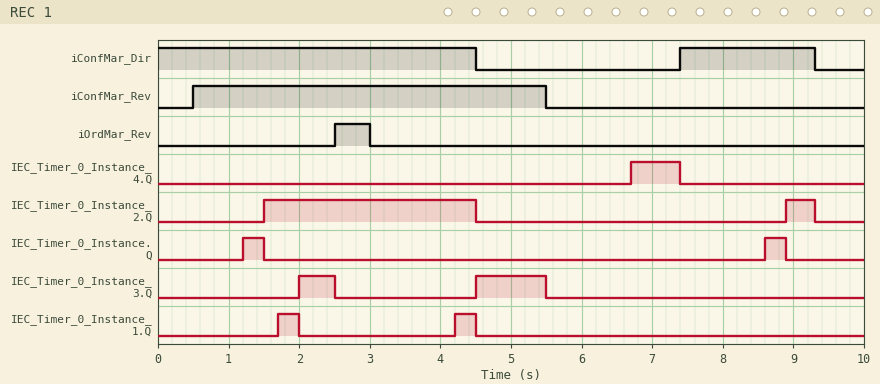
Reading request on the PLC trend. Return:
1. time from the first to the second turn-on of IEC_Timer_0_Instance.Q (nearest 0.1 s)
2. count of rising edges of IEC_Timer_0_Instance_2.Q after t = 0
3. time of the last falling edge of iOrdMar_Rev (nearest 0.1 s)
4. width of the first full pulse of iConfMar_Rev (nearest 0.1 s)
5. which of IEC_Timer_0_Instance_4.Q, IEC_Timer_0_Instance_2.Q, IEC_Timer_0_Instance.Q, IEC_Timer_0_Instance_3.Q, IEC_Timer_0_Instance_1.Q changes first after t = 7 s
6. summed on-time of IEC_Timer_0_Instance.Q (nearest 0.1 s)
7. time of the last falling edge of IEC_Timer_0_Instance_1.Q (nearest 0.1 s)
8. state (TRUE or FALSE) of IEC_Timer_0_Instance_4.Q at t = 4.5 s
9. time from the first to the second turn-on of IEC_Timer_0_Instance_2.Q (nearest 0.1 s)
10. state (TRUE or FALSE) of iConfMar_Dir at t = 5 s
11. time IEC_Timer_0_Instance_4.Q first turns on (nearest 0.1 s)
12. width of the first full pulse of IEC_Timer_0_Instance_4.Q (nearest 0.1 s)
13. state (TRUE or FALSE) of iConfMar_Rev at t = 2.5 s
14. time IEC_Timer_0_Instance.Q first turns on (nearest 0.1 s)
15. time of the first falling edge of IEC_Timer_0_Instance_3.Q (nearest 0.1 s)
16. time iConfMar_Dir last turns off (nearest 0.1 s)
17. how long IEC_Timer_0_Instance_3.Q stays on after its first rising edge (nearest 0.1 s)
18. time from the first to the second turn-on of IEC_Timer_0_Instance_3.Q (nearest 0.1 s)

7.4 s
2
3.0 s
5.0 s
IEC_Timer_0_Instance_4.Q
0.6 s
4.5 s
FALSE
7.4 s
FALSE
6.7 s
0.7 s
TRUE
1.2 s
2.5 s
9.3 s
0.5 s
2.5 s
